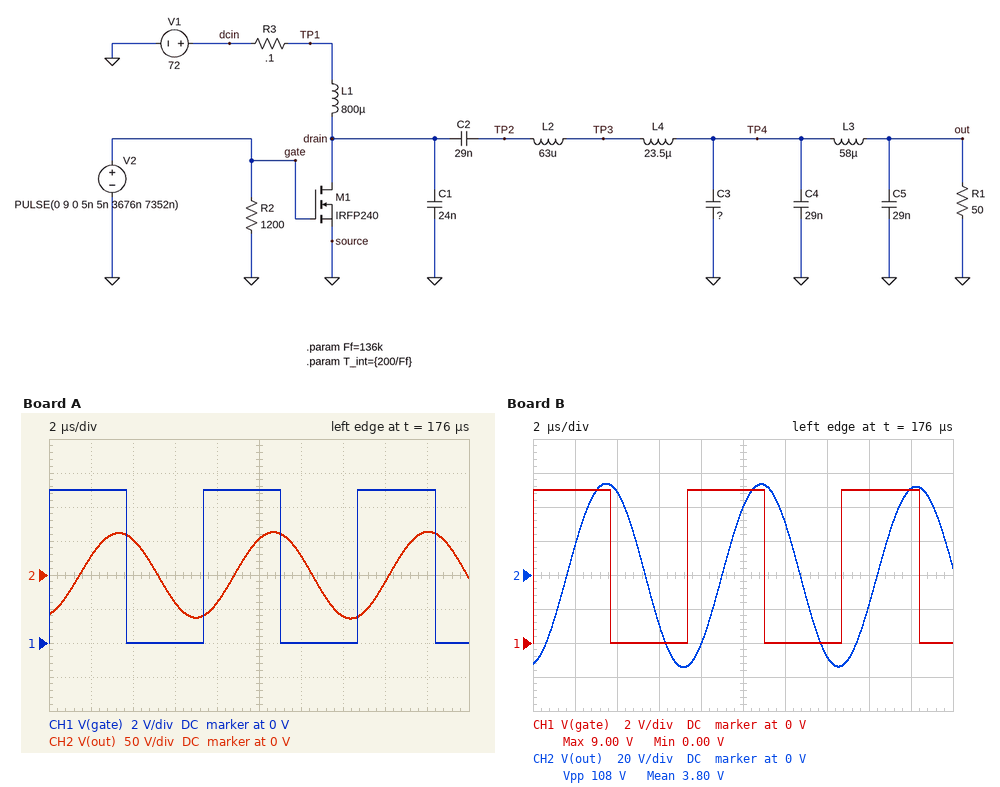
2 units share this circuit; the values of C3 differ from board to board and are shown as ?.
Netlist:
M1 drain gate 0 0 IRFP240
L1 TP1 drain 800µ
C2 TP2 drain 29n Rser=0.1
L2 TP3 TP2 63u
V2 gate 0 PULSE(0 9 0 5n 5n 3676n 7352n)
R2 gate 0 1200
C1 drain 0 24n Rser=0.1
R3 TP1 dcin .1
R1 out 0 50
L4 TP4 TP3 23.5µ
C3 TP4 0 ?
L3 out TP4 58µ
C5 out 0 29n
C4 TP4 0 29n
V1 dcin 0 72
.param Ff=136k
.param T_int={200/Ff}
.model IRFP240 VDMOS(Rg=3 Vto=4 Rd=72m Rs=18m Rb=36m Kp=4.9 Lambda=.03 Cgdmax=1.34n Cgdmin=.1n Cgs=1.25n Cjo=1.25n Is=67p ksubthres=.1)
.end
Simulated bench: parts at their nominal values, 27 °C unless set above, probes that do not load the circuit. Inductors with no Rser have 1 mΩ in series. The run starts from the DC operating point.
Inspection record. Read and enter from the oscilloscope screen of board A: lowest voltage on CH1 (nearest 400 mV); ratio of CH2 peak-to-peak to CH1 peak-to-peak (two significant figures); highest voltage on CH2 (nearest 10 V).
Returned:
0 V
14
60 V
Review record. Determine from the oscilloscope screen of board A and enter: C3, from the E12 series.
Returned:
100 nF
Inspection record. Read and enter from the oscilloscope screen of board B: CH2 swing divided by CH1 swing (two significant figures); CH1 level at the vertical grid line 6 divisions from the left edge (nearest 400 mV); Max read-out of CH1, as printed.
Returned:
12
0 V
9.00 V
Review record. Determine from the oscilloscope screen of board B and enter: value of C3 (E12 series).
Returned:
120 nF
